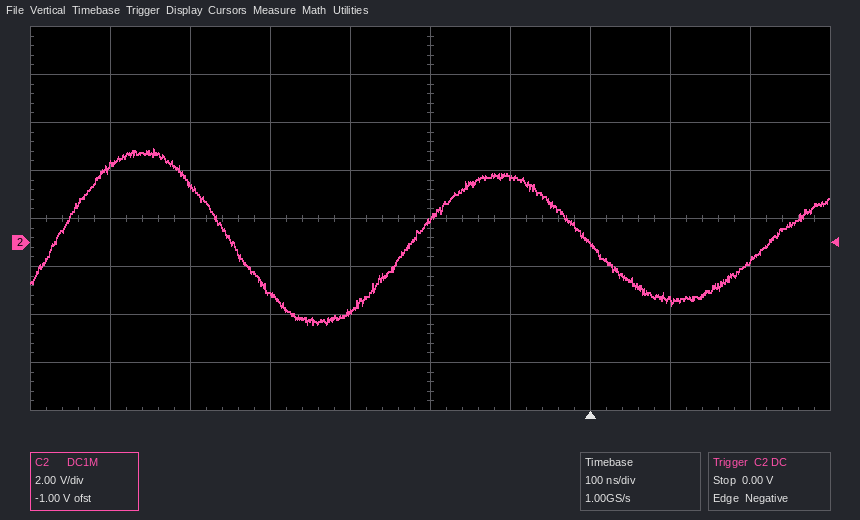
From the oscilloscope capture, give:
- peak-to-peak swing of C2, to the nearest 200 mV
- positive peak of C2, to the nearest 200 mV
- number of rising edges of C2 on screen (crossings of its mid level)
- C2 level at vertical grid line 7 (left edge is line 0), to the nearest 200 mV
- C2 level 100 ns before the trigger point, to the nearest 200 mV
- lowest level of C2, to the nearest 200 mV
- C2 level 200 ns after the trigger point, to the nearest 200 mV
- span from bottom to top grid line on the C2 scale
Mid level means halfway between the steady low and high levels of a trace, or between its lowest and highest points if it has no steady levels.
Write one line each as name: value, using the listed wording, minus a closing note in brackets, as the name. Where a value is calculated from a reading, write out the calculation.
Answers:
peak-to-peak swing of C2, to the nearest 200 mV: 4.0 V − (-3.4 V) = 7.4 V
positive peak of C2, to the nearest 200 mV: 4.0 V
number of rising edges of C2 on screen: 3
C2 level at vertical grid line 7 (left edge is line 0), to the nearest 200 mV: 0.0 V
C2 level 100 ns before the trigger point, to the nearest 200 mV: 2.8 V
lowest level of C2, to the nearest 200 mV: -3.4 V
C2 level 200 ns after the trigger point, to the nearest 200 mV: -800 mV
span from bottom to top grid line on the C2 scale: 16 V
